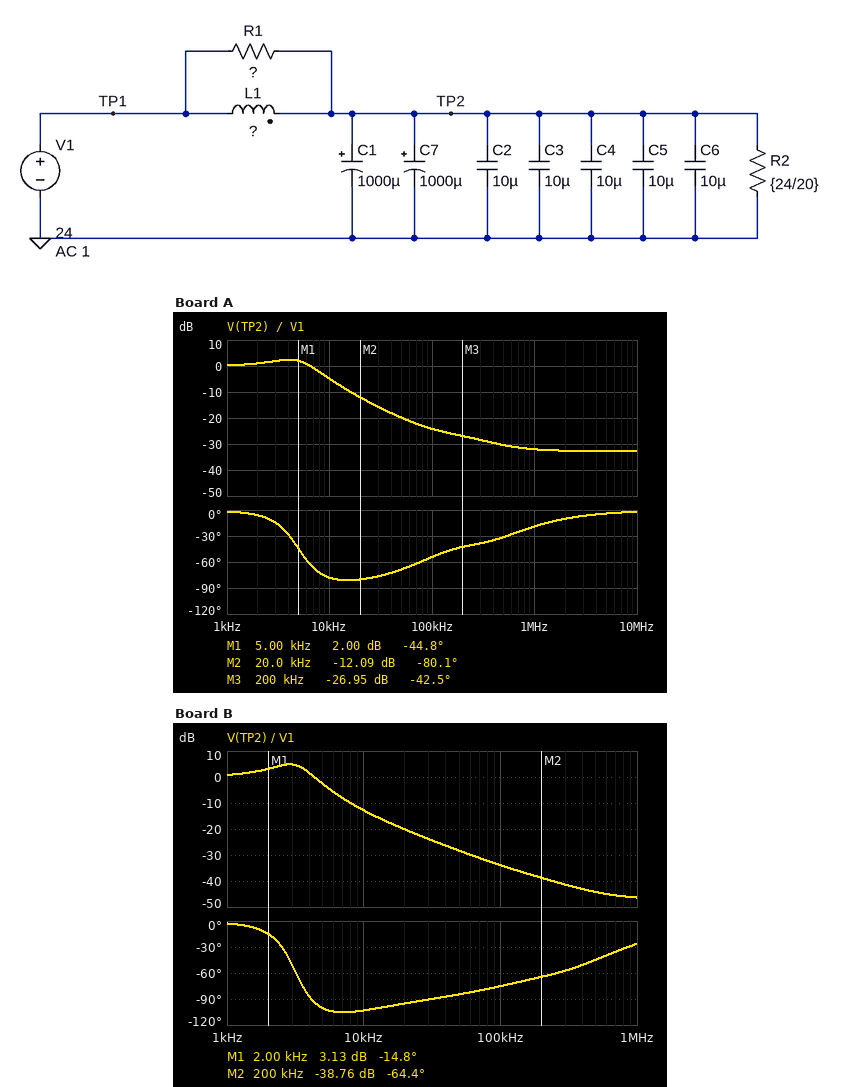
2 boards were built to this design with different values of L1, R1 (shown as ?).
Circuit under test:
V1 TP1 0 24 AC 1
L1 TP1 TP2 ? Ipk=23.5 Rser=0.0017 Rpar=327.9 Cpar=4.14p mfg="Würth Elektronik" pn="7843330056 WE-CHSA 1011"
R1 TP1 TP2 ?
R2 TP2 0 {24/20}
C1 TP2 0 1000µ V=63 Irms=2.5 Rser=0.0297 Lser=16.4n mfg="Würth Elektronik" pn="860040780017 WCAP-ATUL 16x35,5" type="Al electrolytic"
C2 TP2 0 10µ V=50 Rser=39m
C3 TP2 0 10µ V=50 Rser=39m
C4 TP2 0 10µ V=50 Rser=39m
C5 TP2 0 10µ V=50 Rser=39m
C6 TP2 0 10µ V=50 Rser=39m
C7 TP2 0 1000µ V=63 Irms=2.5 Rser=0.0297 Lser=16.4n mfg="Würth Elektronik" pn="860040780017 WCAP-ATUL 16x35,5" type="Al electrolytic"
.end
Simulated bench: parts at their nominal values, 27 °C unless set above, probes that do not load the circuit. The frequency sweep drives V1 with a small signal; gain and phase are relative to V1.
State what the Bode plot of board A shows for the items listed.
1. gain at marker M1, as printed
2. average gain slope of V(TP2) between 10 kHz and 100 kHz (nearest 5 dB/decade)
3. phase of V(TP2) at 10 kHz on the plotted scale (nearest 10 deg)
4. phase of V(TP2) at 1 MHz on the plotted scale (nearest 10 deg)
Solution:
2.00 dB
-20 dB/decade
-80 deg
-20 deg
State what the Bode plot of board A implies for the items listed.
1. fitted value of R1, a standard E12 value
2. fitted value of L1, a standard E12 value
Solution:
0.33 Ω
470 nH
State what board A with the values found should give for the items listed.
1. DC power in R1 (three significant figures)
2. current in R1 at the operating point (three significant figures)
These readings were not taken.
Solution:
3.46 mW
102 mA
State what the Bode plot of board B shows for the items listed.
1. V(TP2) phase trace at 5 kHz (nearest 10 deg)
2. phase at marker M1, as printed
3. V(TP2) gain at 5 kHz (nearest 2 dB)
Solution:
-100 deg
-14.8 deg
-2 dB
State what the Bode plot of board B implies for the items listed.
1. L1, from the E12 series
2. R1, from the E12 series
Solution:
1.2 µH
1.8 Ω
